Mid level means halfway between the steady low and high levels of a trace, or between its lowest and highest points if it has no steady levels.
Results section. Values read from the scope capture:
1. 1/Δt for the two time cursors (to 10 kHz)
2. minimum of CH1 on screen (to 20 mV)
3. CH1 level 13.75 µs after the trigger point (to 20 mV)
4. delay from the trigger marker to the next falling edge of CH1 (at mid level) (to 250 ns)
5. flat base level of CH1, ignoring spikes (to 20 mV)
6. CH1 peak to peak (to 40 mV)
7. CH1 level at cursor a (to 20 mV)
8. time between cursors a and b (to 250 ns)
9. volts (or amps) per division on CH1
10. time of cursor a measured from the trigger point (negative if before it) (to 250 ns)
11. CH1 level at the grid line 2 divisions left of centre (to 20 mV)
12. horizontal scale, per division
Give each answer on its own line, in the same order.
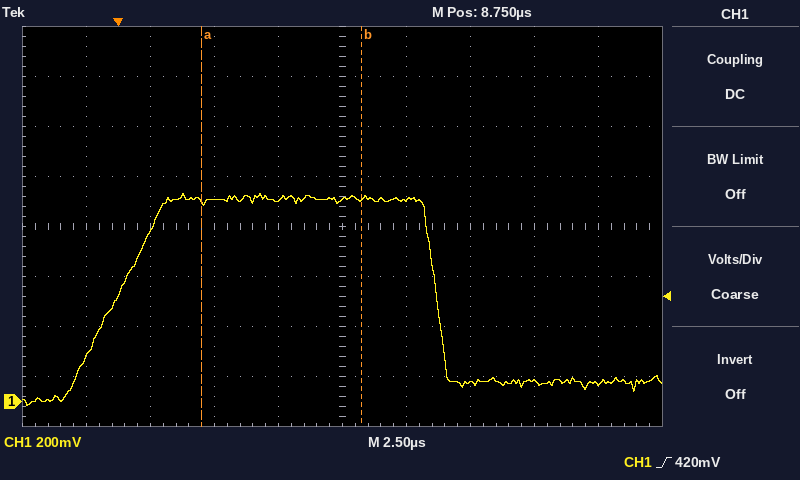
160 kHz
-20 mV
80 mV
12.50 µs
80 mV
840 mV
800 mV
6.25 µs
200 mV
+3.25 µs
800 mV
2.5 µs
